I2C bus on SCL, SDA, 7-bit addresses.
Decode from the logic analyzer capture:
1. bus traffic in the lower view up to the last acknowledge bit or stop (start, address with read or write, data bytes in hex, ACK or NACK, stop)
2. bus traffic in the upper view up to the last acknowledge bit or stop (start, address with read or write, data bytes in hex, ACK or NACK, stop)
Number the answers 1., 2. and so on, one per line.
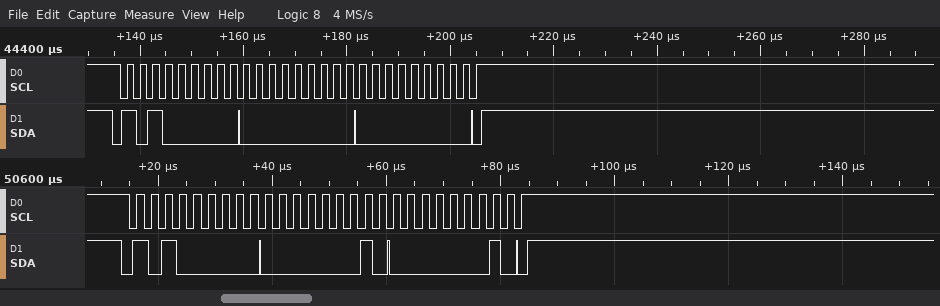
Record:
1. start, address 50 write ACK, 01 ACK, 01 ACK, stop
2. start, address 50 write ACK, 00 ACK, 00 ACK, stop
